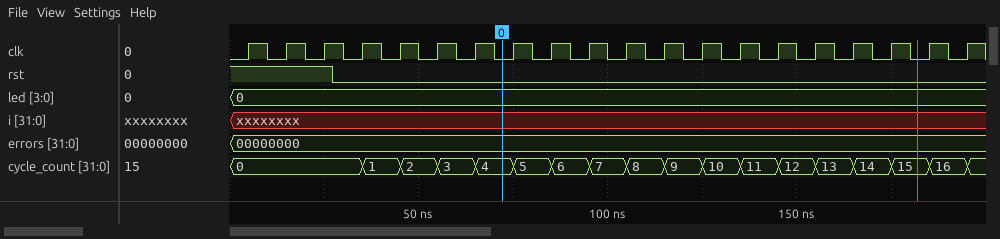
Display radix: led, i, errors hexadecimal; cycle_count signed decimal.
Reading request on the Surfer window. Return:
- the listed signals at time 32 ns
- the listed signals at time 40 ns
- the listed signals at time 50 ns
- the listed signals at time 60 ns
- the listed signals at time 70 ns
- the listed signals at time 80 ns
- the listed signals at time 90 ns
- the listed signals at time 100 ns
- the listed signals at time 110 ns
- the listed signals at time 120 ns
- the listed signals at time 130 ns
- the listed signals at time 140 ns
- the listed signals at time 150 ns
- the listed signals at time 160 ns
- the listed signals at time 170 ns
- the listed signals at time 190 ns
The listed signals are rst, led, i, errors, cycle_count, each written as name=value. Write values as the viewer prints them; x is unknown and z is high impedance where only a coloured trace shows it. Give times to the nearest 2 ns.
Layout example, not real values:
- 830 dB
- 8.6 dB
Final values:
- rst=0, led=0, i=xxxxxxxx, errors=00000000, cycle_count=0
- rst=0, led=0, i=xxxxxxxx, errors=00000000, cycle_count=1
- rst=0, led=0, i=xxxxxxxx, errors=00000000, cycle_count=2
- rst=0, led=0, i=xxxxxxxx, errors=00000000, cycle_count=3
- rst=0, led=0, i=xxxxxxxx, errors=00000000, cycle_count=4
- rst=0, led=0, i=xxxxxxxx, errors=00000000, cycle_count=5
- rst=0, led=0, i=xxxxxxxx, errors=00000000, cycle_count=6
- rst=0, led=0, i=xxxxxxxx, errors=00000000, cycle_count=7
- rst=0, led=0, i=xxxxxxxx, errors=00000000, cycle_count=8
- rst=0, led=0, i=xxxxxxxx, errors=00000000, cycle_count=9
- rst=0, led=0, i=xxxxxxxx, errors=00000000, cycle_count=10
- rst=0, led=0, i=xxxxxxxx, errors=00000000, cycle_count=11
- rst=0, led=0, i=xxxxxxxx, errors=00000000, cycle_count=12
- rst=0, led=0, i=xxxxxxxx, errors=00000000, cycle_count=13
- rst=0, led=0, i=xxxxxxxx, errors=00000000, cycle_count=14
- rst=0, led=0, i=xxxxxxxx, errors=00000000, cycle_count=16
